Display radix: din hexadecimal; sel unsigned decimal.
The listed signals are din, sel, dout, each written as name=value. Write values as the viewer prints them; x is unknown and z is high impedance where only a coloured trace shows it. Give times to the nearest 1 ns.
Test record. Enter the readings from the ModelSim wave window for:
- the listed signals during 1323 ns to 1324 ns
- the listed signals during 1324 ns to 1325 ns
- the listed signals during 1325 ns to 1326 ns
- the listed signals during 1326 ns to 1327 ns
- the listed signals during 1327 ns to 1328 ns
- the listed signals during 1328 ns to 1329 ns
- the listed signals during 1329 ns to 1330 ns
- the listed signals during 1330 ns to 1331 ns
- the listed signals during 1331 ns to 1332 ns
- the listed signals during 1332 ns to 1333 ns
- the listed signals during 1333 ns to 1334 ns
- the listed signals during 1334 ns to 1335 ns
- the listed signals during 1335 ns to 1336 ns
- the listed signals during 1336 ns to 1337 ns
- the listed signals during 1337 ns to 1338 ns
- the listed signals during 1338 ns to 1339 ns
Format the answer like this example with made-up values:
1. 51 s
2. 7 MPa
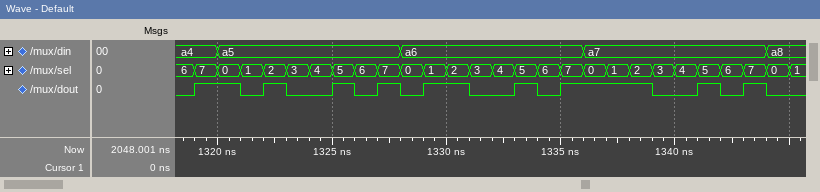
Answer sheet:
1. din=a5, sel=3, dout=0
2. din=a5, sel=4, dout=0
3. din=a5, sel=5, dout=1
4. din=a5, sel=6, dout=0
5. din=a5, sel=7, dout=1
6. din=a6, sel=0, dout=0
7. din=a6, sel=1, dout=1
8. din=a6, sel=2, dout=1
9. din=a6, sel=3, dout=0
10. din=a6, sel=4, dout=0
11. din=a6, sel=5, dout=1
12. din=a6, sel=6, dout=0
13. din=a6, sel=7, dout=1
14. din=a7, sel=0, dout=1
15. din=a7, sel=1, dout=1
16. din=a7, sel=2, dout=1
